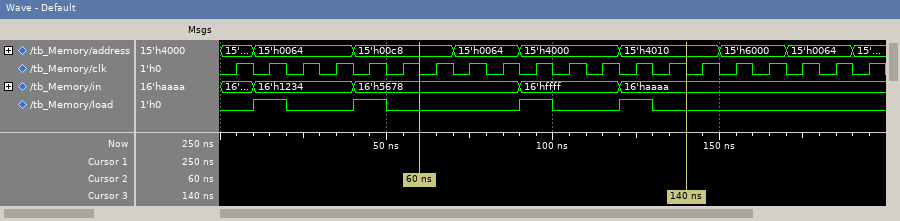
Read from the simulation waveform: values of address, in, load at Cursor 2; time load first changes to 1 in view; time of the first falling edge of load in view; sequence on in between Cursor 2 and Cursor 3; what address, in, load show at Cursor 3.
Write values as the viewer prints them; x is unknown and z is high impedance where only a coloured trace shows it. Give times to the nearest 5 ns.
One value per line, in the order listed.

address=15'h00c8, in=16'h5678, load=0
10 ns
20 ns
16'h5678, 16'hffff, 16'haaaa
address=15'h4010, in=16'haaaa, load=0
